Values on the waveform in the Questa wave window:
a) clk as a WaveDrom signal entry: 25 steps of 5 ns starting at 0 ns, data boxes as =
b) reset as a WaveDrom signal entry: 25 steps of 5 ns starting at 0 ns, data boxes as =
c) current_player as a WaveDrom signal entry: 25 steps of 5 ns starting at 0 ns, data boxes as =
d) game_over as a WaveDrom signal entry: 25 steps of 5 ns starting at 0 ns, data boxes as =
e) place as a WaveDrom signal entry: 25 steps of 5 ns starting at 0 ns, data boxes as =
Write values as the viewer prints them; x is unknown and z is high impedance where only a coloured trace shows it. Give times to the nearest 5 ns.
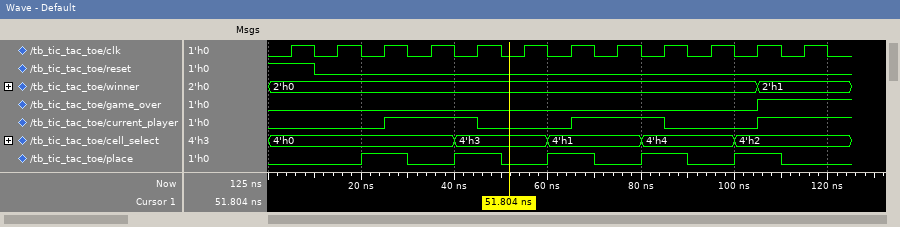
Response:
{name: 'clk', wave: '0101010101010101010101010'}
{name: 'reset', wave: '1.0......................'}
{name: 'current_player', wave: '0....1...0...1...0...1...'}
{name: 'game_over', wave: '0....................1...'}
{name: 'place', wave: '0...1.0.1.0.1.0.1.0.1.0..'}
